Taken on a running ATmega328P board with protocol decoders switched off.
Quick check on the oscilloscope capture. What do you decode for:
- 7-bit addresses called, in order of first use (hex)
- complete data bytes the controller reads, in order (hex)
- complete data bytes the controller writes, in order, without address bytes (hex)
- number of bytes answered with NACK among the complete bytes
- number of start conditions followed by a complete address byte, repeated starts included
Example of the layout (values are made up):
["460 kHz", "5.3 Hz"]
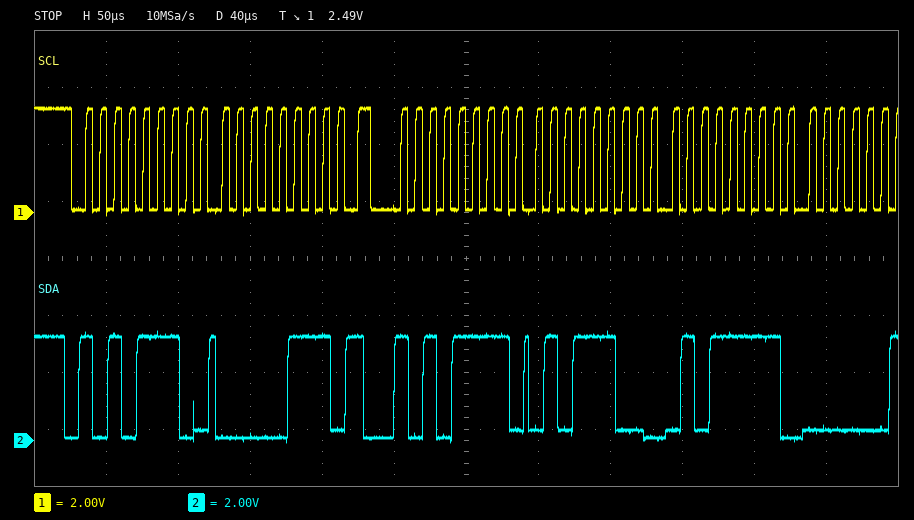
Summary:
["0x57", "5C 5F", "07", "0", "2"]
